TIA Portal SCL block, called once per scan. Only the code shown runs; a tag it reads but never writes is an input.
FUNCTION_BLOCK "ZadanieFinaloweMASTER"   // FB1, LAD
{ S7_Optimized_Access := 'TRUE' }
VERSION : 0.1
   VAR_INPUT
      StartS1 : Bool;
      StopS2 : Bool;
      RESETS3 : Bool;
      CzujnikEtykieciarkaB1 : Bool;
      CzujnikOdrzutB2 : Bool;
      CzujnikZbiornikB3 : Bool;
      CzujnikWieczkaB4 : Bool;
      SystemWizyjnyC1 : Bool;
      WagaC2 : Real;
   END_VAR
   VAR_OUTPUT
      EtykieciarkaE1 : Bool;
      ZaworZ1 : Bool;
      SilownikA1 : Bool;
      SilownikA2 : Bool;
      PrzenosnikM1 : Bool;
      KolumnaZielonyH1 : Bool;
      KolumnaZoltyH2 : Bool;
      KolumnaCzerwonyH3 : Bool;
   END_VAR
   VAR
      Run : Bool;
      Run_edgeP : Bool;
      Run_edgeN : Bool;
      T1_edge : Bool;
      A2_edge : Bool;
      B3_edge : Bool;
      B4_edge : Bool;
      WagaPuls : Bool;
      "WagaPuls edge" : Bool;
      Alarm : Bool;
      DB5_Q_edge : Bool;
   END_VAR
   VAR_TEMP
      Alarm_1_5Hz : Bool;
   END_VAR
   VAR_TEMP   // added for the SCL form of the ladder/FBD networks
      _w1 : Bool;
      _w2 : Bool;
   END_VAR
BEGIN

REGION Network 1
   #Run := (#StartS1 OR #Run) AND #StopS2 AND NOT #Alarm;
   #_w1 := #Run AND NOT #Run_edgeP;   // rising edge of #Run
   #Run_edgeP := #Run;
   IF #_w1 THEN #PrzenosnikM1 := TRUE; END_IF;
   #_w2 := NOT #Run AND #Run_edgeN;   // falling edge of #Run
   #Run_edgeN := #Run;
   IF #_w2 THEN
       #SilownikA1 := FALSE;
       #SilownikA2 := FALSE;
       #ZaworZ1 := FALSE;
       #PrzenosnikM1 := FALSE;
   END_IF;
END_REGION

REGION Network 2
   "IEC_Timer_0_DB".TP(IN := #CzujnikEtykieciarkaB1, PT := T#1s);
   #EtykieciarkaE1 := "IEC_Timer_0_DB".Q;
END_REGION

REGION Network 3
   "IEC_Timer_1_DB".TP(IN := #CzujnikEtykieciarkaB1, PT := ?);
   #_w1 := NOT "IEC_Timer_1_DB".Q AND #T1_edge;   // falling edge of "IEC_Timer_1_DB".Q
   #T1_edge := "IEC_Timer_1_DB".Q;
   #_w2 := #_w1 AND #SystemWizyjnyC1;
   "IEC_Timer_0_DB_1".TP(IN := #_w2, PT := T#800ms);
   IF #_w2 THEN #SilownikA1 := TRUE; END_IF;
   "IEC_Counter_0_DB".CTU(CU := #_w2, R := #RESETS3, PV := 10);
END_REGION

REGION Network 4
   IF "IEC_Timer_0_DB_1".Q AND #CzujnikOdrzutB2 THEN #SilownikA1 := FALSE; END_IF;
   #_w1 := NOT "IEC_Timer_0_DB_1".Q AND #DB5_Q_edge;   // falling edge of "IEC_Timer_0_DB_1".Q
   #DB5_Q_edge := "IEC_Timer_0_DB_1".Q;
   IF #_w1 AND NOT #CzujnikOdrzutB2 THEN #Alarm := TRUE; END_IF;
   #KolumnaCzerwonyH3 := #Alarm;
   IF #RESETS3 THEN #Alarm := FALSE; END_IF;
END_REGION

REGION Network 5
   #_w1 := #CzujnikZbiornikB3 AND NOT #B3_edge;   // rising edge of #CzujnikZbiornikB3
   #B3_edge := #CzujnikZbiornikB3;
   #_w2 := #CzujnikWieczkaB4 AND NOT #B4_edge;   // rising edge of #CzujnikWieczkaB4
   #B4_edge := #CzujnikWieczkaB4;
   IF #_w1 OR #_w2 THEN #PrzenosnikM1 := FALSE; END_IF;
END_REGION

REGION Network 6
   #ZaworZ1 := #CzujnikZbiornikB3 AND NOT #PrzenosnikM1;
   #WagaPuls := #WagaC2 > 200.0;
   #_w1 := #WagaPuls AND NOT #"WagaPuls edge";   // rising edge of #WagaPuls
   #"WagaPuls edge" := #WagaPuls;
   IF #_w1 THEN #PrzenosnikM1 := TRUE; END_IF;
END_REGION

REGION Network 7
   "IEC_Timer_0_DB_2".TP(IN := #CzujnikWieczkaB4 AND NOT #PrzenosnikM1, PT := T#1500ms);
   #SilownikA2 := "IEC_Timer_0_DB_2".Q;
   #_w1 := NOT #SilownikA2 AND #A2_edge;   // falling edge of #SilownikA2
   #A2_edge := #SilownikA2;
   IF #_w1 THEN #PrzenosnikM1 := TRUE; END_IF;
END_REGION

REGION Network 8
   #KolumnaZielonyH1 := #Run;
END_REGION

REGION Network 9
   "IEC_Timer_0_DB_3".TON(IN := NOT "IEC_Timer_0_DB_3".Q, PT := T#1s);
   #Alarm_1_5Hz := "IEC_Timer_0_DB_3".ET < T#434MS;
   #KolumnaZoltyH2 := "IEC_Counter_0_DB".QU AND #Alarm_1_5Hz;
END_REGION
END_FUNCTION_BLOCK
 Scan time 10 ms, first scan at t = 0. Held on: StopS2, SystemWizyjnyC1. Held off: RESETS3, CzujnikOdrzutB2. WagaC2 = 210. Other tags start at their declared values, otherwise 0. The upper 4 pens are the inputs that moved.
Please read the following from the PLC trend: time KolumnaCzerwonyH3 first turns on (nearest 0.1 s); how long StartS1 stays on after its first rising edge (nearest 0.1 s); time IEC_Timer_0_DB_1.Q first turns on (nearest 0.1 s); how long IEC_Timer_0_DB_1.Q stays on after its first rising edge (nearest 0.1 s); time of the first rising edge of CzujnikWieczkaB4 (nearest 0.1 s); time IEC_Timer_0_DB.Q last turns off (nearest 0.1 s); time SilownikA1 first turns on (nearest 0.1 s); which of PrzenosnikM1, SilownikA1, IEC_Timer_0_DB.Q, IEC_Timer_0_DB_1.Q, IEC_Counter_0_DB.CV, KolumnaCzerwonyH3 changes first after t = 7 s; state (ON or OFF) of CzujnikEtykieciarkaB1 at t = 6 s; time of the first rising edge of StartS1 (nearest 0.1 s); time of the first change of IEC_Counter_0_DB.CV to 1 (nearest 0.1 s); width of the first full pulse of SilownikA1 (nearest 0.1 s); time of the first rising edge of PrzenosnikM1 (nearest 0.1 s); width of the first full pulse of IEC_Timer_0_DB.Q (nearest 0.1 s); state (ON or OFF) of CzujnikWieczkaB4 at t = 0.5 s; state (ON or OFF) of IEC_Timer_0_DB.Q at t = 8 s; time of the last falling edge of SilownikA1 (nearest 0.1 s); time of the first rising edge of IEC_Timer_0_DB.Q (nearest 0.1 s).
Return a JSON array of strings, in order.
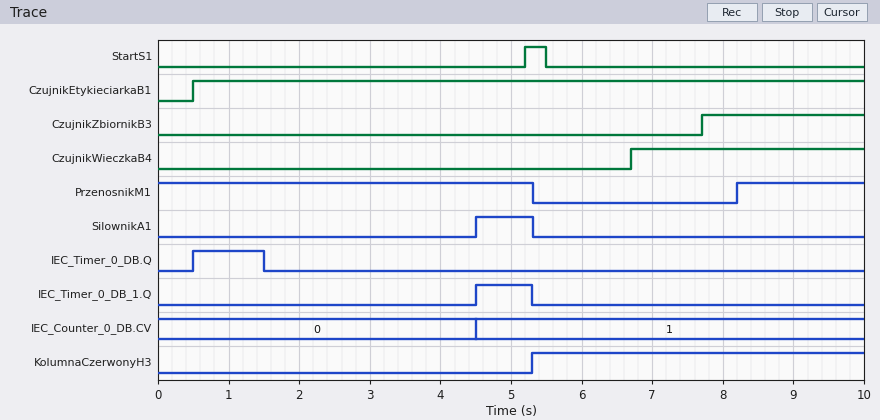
["5.3 s", "0.3 s", "4.5 s", "0.8 s", "6.7 s", "1.5 s", "4.5 s", "PrzenosnikM1", "ON", "5.2 s", "4.5 s", "0.8 s", "8.2 s", "1.0 s", "OFF", "OFF", "5.3 s", "0.5 s"]
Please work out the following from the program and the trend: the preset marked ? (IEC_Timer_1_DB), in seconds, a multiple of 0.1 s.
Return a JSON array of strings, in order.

["4.0 s"]
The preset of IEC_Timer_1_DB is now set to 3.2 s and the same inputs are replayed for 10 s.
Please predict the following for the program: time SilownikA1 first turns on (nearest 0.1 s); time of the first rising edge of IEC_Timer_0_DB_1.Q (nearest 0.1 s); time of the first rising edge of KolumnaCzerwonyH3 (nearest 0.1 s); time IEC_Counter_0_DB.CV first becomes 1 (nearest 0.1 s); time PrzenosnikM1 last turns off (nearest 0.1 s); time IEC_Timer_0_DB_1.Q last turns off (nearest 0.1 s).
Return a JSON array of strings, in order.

["3.7 s", "3.7 s", "4.5 s", "3.7 s", "6.7 s", "4.5 s"]
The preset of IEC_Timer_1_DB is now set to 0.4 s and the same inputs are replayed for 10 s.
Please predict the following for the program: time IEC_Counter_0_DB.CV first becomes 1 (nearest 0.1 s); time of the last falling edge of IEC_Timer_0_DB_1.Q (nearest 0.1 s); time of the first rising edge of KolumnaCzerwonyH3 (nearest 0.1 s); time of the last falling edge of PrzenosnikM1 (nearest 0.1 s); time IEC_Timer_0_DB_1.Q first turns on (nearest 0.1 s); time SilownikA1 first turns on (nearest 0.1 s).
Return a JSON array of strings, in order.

["0.9 s", "1.7 s", "1.7 s", "6.7 s", "0.9 s", "0.9 s"]
